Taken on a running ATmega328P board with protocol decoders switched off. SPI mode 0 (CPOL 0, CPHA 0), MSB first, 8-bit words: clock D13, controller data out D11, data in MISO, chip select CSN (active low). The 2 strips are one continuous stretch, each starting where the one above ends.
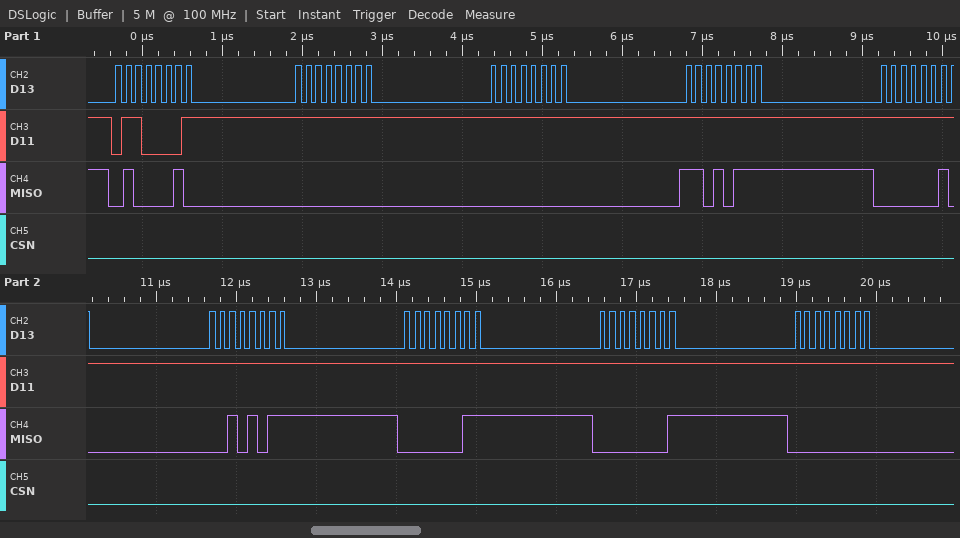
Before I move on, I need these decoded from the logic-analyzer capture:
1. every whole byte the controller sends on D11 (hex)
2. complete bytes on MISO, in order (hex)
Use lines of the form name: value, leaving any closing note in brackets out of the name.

every whole byte the controller sends on D11: 61 FF FF FF FF FF FF FF FF
complete bytes on MISO, in order: 42 00 00 D7 02 2B 03 01 00
